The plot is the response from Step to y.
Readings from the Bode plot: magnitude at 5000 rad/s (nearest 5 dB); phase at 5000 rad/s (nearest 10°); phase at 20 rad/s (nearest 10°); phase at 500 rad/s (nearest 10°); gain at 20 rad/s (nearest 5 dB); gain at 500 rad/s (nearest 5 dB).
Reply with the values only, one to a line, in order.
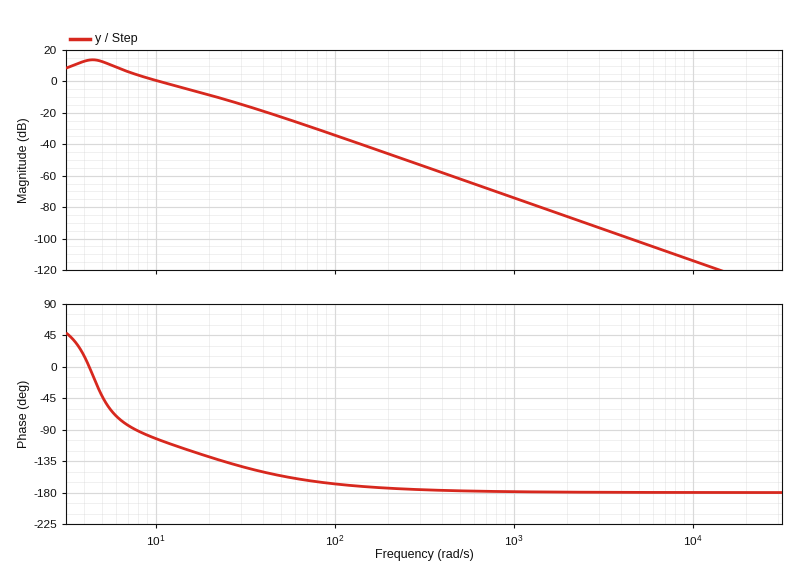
-100 dB
-180°
-130°
-180°
-10 dB
-60 dB
